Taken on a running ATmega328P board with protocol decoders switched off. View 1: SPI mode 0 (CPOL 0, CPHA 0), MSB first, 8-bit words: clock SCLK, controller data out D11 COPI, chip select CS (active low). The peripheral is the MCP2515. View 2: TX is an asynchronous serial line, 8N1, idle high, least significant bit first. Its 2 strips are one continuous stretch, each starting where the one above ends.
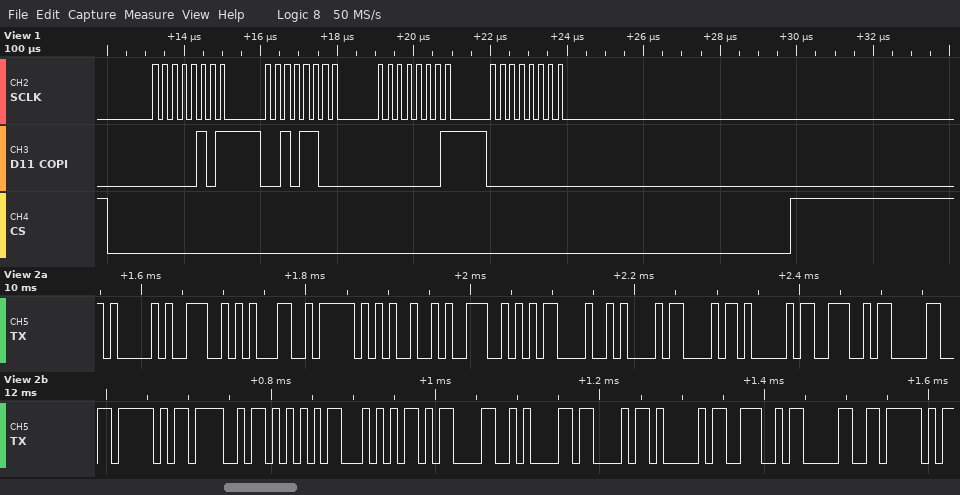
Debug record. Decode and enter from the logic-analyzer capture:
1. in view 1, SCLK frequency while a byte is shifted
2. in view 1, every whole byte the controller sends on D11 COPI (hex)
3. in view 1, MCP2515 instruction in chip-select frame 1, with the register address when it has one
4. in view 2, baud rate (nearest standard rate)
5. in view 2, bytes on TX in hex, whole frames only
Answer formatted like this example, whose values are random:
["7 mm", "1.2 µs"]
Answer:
["4 MHz", "05 2C 01 00", "BIT MODIFY 0x2C", "115200 baud", "0x41 0x4E 0x31 0x5F 0x49 0x4E 0x0D 0x0A 0x43 0x41 0x4E 0x30 0x5F 0x4F 0x55 0x54 0x0D 0x0A 0x43 0x41 0x4E 0x30 0x5F"]
